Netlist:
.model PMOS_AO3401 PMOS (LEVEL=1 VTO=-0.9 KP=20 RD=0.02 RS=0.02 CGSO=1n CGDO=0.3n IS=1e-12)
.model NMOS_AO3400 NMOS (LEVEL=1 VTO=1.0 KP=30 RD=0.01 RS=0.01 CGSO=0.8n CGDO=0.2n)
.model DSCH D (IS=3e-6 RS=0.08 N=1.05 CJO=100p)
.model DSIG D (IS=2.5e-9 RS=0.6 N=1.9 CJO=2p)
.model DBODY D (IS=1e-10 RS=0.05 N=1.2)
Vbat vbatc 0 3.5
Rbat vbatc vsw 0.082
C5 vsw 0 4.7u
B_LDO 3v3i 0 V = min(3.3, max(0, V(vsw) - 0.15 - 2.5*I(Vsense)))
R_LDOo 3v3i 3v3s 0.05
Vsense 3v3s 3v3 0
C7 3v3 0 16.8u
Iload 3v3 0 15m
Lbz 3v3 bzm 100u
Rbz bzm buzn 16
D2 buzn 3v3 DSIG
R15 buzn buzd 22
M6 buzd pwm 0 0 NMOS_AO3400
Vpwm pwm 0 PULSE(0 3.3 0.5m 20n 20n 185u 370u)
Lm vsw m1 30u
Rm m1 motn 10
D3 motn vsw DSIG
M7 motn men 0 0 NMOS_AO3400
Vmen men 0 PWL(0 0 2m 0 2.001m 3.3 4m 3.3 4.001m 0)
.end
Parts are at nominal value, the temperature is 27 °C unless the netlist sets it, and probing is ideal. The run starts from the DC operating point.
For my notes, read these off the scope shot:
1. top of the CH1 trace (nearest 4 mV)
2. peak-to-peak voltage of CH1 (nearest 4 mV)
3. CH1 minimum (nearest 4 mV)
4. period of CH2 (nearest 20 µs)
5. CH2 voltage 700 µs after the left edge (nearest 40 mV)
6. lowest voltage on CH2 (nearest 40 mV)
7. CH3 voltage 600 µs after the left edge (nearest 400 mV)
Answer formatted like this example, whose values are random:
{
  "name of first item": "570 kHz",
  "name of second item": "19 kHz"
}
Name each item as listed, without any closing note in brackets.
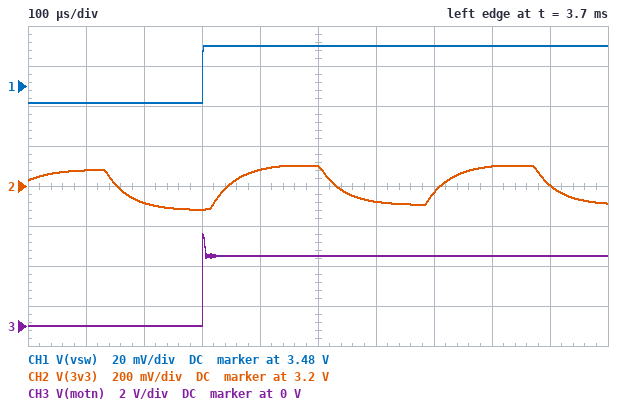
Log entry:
{
  "top of the CH1 trace": "3.500 V",
  "peak-to-peak voltage of CH1": "28 mV",
  "CH1 minimum": "3.472 V",
  "period of CH2": "360 µs",
  "CH2 voltage 700 µs after the left edge": "3.16 V",
  "lowest voltage on CH2": "3.08 V",
  "CH3 voltage 600 µs after the left edge": "3.6 V"
}
